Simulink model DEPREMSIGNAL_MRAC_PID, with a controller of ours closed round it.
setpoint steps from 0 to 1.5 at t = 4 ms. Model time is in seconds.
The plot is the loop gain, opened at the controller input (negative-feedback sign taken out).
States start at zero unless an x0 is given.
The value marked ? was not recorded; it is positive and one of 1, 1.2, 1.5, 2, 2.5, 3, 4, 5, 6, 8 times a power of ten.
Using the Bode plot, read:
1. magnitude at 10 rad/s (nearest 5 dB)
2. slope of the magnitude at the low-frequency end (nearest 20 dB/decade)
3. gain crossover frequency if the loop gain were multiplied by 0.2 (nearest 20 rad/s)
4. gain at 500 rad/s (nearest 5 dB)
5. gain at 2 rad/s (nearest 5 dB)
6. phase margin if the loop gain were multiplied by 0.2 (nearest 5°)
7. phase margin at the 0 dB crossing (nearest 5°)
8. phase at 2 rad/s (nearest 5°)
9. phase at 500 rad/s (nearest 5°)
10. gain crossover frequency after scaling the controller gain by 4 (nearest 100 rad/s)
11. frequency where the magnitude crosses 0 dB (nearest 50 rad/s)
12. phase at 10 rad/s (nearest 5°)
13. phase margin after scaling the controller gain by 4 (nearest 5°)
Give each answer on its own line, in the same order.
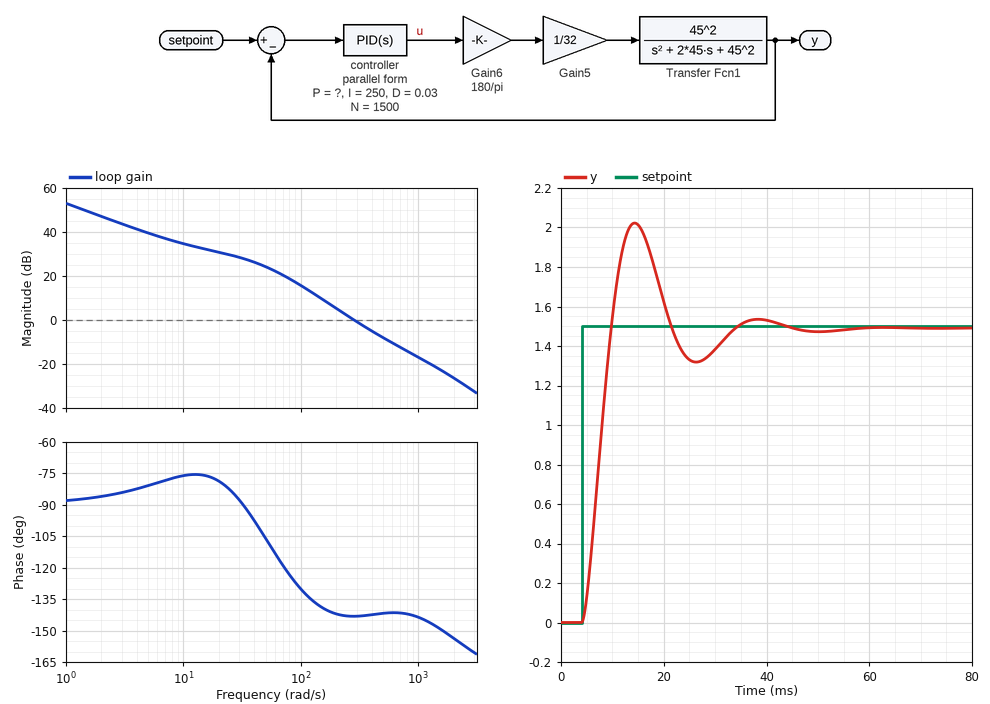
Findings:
35 dB
-20 dB/decade
120 rad/s
-10 dB
45 dB
45°
35°
-85°
-140°
700 rad/s
300 rad/s
-75°
40°
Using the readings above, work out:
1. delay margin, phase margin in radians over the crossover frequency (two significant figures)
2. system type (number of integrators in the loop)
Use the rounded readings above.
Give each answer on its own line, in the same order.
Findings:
0.0020 s
1
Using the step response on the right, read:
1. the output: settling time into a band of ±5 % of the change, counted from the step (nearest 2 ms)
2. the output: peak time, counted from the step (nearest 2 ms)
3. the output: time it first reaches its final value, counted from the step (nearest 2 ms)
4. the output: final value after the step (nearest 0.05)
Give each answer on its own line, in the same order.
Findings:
28 ms
10 ms
6 ms
1.50
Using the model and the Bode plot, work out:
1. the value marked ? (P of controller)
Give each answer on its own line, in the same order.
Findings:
20
